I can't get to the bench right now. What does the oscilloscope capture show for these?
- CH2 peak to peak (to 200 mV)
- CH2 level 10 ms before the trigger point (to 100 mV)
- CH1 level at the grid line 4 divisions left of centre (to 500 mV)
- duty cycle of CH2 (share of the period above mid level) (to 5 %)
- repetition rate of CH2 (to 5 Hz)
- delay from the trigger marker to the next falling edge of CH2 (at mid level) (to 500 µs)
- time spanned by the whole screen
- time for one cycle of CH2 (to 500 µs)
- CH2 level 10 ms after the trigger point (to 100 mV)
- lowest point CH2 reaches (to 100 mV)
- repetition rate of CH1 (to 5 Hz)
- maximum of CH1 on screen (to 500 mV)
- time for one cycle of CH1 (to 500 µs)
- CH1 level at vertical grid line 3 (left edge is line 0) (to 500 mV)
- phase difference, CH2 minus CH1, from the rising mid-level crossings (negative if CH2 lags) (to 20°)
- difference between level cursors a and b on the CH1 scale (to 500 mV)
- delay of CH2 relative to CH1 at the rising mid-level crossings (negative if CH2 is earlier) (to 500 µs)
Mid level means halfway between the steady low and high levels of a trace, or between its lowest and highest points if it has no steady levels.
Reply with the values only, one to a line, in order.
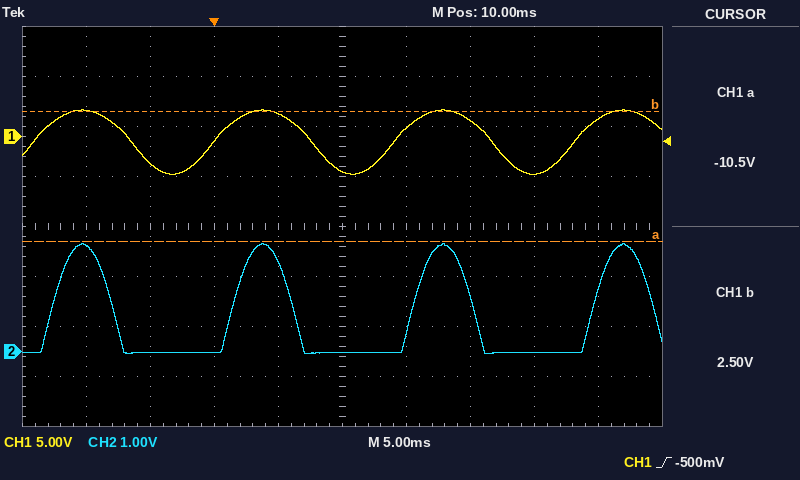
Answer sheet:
2.2 V
2.1 V
2.5 V
30 %
70 Hz
6.0 ms
50 ms
14.0 ms
0.0 V
0.0 V
70 Hz
2.5 V
14.0 ms
-500 mV
-40°
13.0 V
+1.5 ms
